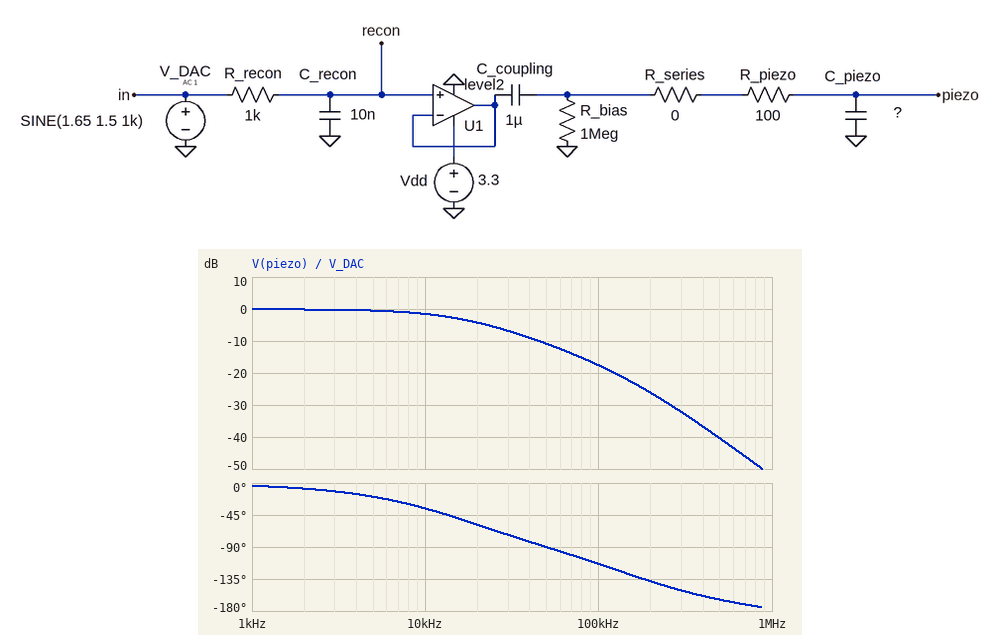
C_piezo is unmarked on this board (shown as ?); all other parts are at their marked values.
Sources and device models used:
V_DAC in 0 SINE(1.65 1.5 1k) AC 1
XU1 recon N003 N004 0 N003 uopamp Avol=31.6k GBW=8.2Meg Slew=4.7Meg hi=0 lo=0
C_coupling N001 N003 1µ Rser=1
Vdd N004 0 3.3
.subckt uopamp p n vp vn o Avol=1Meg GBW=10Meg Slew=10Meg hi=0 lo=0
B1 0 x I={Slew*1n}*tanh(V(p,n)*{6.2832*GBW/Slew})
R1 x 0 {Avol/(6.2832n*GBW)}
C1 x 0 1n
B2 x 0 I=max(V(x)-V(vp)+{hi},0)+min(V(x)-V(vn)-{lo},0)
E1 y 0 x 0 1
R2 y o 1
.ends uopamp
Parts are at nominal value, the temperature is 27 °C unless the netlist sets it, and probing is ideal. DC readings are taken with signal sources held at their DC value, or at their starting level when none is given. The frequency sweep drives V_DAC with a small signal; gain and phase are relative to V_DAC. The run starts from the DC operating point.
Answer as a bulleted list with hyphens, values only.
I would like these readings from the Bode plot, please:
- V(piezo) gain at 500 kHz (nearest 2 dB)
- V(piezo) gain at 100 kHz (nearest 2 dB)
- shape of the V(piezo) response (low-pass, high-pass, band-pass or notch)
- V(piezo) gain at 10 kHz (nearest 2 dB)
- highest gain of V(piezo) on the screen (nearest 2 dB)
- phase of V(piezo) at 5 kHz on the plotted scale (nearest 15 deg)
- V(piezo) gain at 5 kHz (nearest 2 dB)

- -40 dB
- -18 dB
- low-pass
- -2 dB
- 0 dB
- -15 deg
- 0 dB
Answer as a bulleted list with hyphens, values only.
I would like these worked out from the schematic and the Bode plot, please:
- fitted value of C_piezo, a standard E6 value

- 10 nF
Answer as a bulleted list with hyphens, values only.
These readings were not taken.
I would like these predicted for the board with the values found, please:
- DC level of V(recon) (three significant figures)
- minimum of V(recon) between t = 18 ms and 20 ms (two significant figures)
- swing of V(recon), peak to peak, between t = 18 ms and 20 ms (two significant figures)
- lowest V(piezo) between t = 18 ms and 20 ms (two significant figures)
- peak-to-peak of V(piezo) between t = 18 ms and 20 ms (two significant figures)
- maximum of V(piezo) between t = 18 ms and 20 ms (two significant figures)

- 1.65 V
- 150 mV
- 3.0 V
- -1.5 V
- 3.0 V
- 1.5 V
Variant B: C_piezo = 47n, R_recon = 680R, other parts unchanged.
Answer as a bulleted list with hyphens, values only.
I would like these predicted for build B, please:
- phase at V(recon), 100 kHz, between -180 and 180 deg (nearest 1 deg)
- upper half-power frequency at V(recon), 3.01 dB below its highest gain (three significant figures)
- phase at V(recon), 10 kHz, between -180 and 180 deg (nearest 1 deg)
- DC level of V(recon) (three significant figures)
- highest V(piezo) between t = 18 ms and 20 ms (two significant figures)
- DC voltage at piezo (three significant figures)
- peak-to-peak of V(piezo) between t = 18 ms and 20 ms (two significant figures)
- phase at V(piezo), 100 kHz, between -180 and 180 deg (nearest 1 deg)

- -77 deg
- 23.4 kHz
- -23 deg
- 1.65 V
- 1.4 V
- 1.39 V
- 2.9 V
- -148 deg
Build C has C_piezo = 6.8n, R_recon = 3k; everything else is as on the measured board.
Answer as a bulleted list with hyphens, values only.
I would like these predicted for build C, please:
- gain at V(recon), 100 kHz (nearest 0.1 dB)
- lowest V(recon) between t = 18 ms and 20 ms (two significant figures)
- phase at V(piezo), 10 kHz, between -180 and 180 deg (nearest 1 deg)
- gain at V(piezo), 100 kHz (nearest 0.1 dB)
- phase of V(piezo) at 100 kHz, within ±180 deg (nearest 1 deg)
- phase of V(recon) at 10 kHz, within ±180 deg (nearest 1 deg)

- -25.5 dB
- 180 mV
- -65 deg
- -26.3 dB
- -111 deg
- -62 deg
